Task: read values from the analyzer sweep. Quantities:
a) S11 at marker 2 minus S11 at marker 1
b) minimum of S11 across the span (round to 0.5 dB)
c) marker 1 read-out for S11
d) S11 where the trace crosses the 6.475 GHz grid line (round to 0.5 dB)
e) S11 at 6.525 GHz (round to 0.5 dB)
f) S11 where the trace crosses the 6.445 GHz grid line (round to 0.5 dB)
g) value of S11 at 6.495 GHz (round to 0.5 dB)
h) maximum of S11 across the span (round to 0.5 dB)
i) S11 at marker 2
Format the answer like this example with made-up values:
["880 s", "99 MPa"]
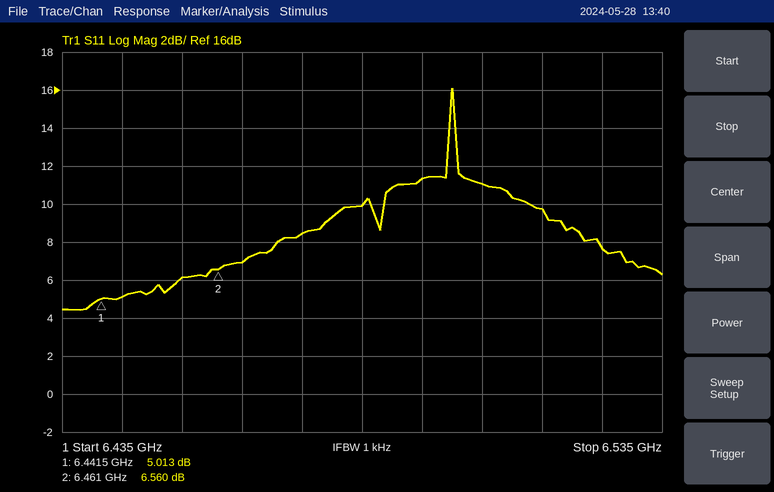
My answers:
["1.547 dB", "4.5 dB", "5.013 dB", "8.5 dB", "7.5 dB", "5.0 dB", "11.5 dB", "16.0 dB", "6.560 dB"]
